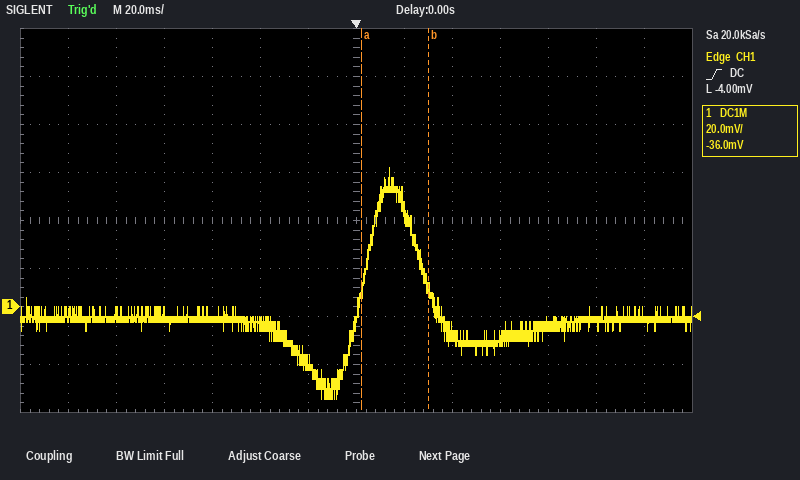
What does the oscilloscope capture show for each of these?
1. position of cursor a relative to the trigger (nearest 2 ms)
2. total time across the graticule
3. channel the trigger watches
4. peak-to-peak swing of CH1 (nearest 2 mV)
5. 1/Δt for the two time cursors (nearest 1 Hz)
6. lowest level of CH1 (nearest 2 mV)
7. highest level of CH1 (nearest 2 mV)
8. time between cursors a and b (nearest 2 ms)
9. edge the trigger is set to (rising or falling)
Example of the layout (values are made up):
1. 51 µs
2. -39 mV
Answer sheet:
1. +2 ms
2. 280 ms
3. CH1
4. 96 mV
5. 36 Hz
6. -38 mV
7. 58 mV
8. 28 ms
9. rising
